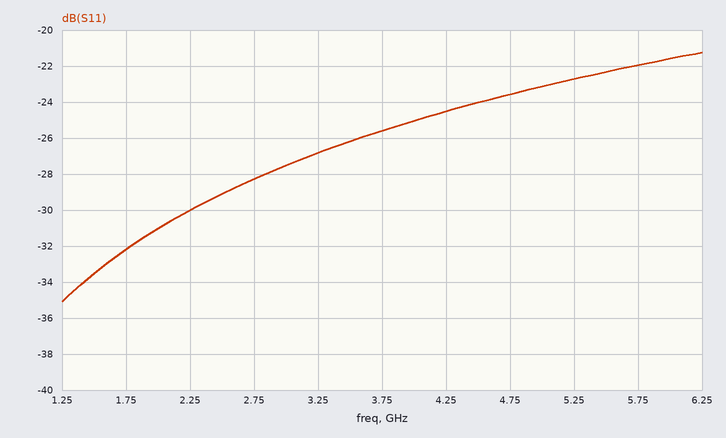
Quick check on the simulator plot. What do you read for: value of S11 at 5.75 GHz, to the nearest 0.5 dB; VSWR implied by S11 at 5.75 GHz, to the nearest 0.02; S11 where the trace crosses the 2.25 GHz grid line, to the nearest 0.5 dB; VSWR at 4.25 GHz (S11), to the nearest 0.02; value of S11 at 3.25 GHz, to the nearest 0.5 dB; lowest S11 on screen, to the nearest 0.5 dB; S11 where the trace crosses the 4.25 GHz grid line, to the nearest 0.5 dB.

-22.0 dB
1.18
-30.0 dB
1.12
-27.0 dB
-35.0 dB
-24.5 dB
